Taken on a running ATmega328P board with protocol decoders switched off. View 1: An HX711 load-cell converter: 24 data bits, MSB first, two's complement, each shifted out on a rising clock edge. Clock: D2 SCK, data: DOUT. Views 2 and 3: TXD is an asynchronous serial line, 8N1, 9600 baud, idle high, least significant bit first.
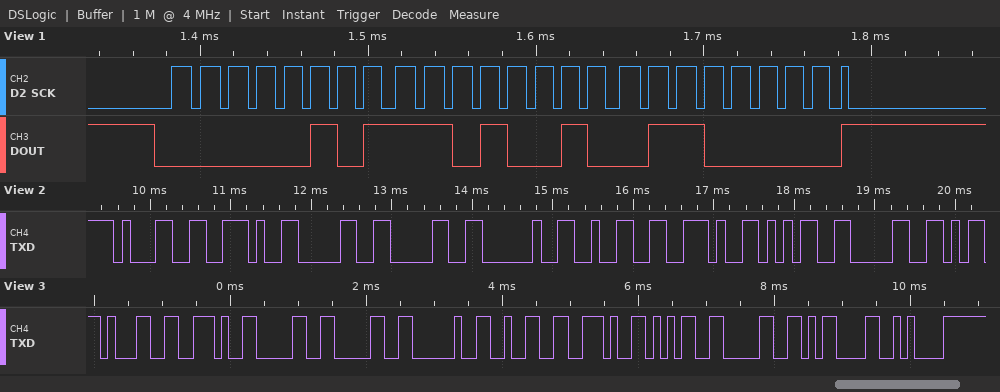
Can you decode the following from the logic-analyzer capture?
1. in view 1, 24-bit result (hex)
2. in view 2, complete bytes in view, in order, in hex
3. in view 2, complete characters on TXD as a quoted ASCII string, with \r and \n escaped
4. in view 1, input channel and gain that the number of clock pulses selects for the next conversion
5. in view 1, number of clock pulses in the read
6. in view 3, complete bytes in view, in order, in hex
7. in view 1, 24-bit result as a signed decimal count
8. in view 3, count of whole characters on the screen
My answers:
0x05D260
31 2E 30 30 20 32 2E 35 30
"1.00 2.50"
channel A, gain 128
25
31 2E 30 30 20 32 2E 35 30 0D 0A
381536
11
